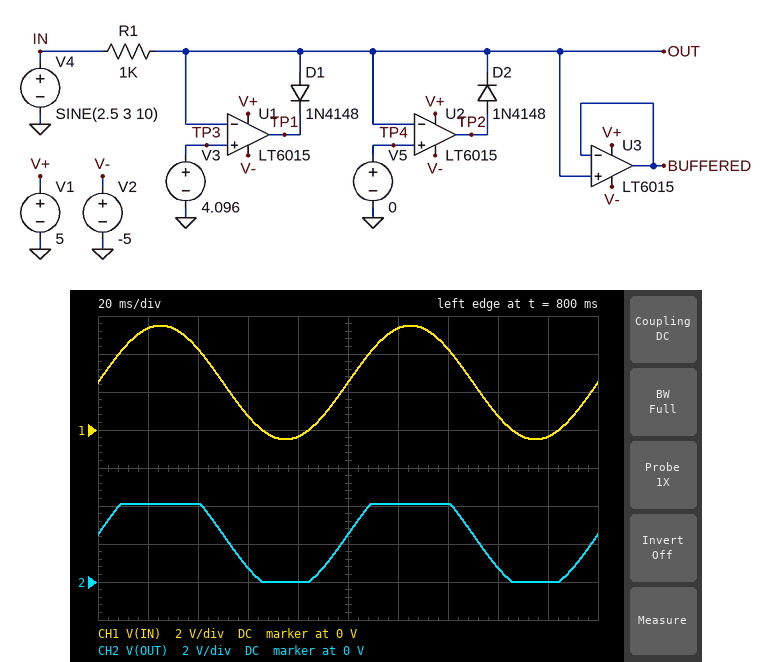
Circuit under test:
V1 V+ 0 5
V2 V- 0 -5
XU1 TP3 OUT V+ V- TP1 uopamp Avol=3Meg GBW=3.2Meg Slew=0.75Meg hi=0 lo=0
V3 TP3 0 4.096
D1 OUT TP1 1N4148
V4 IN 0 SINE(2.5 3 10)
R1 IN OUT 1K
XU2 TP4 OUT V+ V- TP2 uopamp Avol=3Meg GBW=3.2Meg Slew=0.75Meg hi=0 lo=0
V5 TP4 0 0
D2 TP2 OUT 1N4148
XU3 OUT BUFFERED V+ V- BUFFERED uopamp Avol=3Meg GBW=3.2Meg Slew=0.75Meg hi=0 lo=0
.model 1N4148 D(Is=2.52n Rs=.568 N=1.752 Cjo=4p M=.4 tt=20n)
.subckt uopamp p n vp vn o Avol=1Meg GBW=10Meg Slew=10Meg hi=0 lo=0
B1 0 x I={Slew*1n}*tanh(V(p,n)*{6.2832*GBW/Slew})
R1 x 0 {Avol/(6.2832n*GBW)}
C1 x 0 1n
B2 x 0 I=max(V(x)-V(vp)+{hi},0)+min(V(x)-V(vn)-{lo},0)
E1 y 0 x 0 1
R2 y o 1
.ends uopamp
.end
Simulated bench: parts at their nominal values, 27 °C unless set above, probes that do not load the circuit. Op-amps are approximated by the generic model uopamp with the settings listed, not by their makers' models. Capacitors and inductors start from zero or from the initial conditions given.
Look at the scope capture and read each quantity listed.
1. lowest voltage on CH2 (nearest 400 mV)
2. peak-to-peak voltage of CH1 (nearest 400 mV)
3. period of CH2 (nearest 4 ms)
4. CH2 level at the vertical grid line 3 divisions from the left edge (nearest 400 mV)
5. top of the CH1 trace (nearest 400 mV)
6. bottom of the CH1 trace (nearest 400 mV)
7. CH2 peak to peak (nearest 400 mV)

0 V
6.0 V
100 ms
800 mV
5.6 V
-400 mV
4.0 V
